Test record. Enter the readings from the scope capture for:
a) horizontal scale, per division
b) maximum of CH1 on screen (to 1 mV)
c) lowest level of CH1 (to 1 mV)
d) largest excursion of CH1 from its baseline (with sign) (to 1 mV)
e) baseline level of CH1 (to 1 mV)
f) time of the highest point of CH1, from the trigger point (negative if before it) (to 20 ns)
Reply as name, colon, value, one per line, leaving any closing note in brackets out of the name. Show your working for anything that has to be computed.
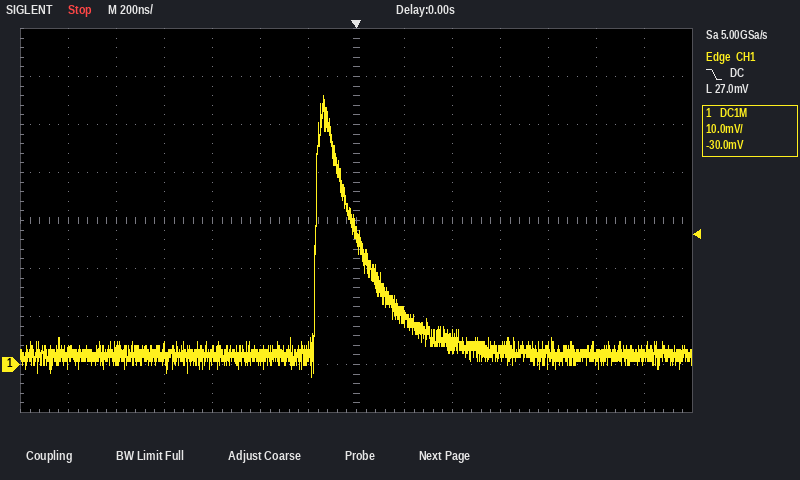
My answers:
horizontal scale, per division: 200 ns
maximum of CH1 on screen: 56 mV
lowest level of CH1: -2 mV
largest excursion of CH1 from its baseline (with sign): 56 mV − (2 mV) = +54 mV
baseline level of CH1: 2 mV
time of the highest point of CH1, from the trigger point (negative if before it): -140 ns
